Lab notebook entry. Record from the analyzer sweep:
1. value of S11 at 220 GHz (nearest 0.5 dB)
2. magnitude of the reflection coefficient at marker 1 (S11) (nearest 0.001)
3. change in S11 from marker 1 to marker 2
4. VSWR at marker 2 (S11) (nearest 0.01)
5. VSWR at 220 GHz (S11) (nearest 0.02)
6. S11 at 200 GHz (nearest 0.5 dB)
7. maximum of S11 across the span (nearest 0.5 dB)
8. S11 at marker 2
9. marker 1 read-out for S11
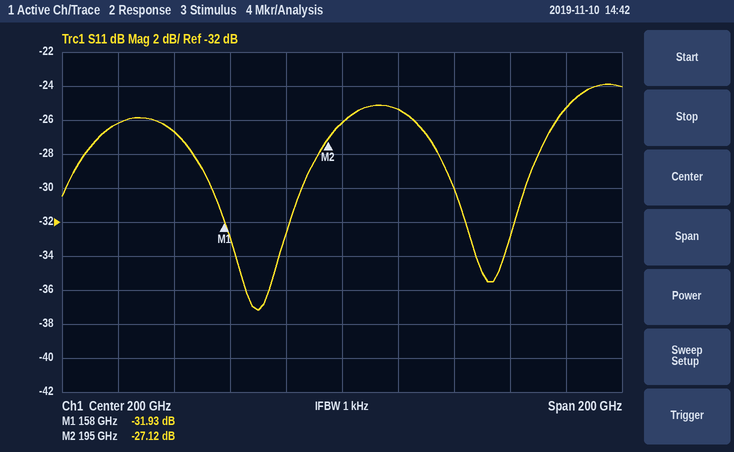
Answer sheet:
-25.5 dB
0.025
4.81 dB
1.09
1.12
-26.0 dB
-24.0 dB
-27.12 dB
-31.93 dB
